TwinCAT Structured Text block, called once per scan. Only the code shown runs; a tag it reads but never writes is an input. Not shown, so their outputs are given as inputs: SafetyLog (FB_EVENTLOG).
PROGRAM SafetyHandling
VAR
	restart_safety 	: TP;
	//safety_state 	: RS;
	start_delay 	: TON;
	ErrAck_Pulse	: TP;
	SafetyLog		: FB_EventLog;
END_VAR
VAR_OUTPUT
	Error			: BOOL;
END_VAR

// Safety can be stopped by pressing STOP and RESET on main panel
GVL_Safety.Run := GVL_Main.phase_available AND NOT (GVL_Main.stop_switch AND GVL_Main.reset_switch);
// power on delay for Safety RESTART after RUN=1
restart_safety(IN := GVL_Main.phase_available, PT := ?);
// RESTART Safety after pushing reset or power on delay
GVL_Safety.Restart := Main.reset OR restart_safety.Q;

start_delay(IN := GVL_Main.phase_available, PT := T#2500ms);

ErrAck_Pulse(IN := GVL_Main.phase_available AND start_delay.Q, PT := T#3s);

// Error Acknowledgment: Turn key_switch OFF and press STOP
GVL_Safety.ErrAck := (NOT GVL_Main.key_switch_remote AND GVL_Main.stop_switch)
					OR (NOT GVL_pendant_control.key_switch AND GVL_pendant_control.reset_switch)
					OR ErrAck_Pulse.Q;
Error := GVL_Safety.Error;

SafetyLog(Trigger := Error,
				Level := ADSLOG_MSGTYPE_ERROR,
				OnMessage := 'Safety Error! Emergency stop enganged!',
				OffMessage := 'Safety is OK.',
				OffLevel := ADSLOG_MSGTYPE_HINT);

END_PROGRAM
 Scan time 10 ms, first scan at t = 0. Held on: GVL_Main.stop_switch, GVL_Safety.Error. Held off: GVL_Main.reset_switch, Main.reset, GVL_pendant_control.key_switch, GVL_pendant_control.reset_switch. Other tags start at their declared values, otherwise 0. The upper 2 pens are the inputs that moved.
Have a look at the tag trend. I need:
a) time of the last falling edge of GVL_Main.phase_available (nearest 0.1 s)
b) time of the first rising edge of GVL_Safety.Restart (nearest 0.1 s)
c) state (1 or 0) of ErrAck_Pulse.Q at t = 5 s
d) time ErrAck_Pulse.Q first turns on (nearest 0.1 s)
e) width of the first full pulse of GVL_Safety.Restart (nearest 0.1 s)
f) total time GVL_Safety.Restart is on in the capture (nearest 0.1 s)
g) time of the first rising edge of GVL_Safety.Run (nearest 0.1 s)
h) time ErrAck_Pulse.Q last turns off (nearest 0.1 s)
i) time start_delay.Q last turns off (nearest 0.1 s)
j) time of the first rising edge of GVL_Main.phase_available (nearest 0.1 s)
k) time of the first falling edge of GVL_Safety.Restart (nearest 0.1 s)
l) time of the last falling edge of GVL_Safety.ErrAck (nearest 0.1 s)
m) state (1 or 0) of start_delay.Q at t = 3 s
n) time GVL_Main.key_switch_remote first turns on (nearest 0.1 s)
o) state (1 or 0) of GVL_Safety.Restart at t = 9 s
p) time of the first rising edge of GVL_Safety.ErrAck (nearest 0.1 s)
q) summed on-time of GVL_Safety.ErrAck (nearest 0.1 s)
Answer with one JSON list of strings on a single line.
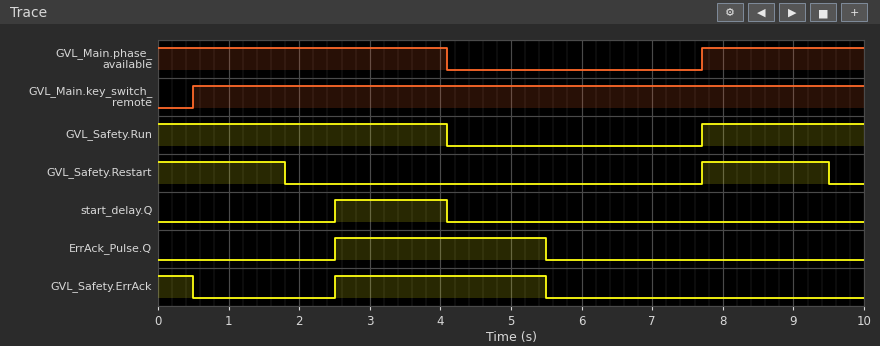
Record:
["4.1 s", "7.7 s", "1", "2.5 s", "1.8 s", "3.6 s", "7.7 s", "5.5 s", "4.1 s", "7.7 s", "1.8 s", "5.5 s", "1", "0.5 s", "1", "2.5 s", "3.5 s"]
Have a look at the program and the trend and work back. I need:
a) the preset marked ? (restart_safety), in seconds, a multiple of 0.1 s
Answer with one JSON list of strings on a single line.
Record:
["1.8 s"]
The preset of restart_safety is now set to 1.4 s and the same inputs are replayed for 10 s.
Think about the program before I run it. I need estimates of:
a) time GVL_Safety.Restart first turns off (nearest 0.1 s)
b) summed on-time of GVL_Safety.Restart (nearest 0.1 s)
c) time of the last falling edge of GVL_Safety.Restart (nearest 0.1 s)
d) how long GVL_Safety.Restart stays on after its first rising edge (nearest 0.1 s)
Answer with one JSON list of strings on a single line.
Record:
["1.4 s", "2.8 s", "9.1 s", "1.4 s"]
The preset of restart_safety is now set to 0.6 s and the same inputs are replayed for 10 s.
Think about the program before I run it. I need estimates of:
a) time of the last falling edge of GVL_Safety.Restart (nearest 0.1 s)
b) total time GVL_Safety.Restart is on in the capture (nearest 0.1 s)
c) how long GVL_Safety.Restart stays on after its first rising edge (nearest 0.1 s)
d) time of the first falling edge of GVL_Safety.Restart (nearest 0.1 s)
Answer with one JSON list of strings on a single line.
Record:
["8.3 s", "1.2 s", "0.6 s", "0.6 s"]
